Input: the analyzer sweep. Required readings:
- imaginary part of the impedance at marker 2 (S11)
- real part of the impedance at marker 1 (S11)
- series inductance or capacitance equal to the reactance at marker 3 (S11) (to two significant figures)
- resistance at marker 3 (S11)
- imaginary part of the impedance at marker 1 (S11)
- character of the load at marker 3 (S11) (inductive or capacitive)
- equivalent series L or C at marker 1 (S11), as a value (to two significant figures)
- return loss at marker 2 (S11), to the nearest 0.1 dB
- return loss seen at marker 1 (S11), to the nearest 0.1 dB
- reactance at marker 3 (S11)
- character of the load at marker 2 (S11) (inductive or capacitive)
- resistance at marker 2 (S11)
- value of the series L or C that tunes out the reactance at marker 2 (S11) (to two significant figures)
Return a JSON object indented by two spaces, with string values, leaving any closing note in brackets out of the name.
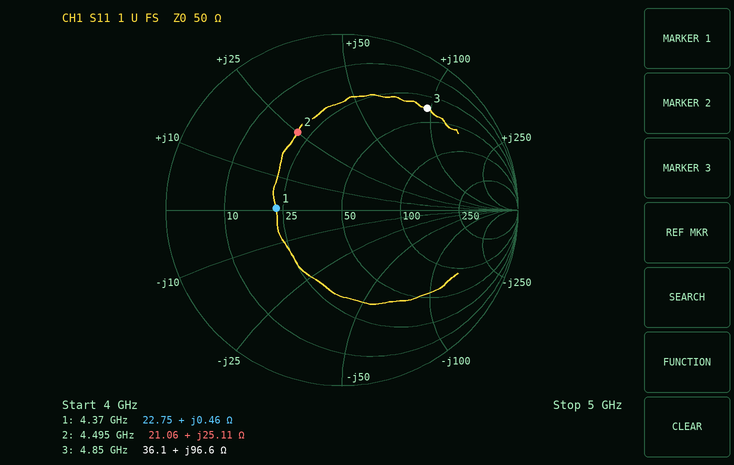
{
  "imaginary part of the impedance at marker 2": "+25.11 Ω",
  "real part of the impedance at marker 1": "22.75 Ω",
  "series inductance or capacitance equal to the reactance at marker 3 (S11)": "3.2 nH",
  "resistance at marker 3": "36.1 Ω",
  "imaginary part of the impedance at marker 1": "+0.46 Ω",
  "character of the load at marker 3 (S11)": "inductive",
  "equivalent series L or C at marker 1 (S11), as a value": "17 pH",
  "return loss at marker 2 (S11), to the nearest 0.1 dB": "5.9 dB",
  "return loss seen at marker 1 (S11), to the nearest 0.1 dB": "8.5 dB",
  "reactance at marker 3": "+96.6 Ω",
  "character of the load at marker 2 (S11)": "inductive",
  "resistance at marker 2": "21.06 Ω",
  "value of the series L or C that tunes out the reactance at marker 2 (S11)": "1.4 pF"
}
